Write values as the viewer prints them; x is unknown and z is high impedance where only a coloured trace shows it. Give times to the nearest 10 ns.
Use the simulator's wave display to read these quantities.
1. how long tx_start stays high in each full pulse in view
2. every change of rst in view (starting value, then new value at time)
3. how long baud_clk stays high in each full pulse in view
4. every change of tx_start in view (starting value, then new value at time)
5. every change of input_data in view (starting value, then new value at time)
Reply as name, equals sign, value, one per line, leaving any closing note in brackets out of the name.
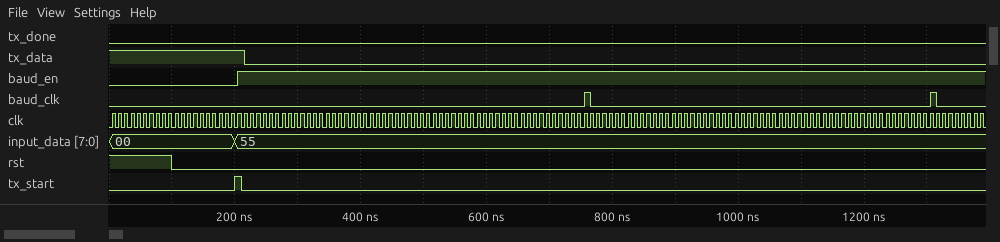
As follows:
how long tx_start stays high in each full pulse in view = 10 ns
every change of rst in view = 1, 0 at 100 ns
how long baud_clk stays high in each full pulse in view = 10 ns, 10 ns
every change of tx_start in view = 0, 1 at 200 ns, 0 at 210 ns
every change of input_data in view = 00, 55 at 200 ns
